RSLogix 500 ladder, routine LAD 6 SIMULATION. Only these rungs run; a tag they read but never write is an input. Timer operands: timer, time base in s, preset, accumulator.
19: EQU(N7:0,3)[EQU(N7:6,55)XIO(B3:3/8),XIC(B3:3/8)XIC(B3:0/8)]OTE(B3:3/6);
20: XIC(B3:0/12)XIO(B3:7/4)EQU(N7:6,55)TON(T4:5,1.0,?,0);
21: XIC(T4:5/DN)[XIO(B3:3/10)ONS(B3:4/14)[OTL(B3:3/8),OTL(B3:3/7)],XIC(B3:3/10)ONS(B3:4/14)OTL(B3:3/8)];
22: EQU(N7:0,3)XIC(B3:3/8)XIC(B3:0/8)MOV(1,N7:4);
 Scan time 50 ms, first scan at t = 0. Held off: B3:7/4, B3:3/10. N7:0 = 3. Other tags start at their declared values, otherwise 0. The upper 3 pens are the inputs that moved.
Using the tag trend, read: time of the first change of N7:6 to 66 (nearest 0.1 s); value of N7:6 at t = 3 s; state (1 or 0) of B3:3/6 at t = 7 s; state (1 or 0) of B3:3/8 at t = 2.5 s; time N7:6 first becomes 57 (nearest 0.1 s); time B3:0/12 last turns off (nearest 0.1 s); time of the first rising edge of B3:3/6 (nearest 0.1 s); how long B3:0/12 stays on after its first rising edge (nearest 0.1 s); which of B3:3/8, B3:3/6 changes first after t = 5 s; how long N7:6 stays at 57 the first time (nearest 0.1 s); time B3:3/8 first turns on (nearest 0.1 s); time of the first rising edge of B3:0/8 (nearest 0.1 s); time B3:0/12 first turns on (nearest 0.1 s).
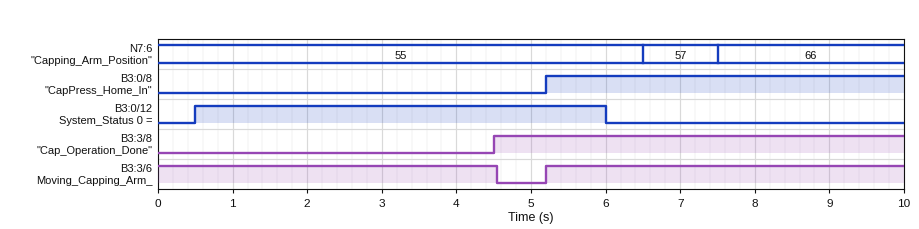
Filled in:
7.5 s
55
1
0
6.5 s
6.0 s
5.2 s
5.5 s
B3:3/6
1.0 s
4.5 s
5.2 s
0.5 s
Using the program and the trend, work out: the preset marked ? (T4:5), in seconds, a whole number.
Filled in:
4 s
